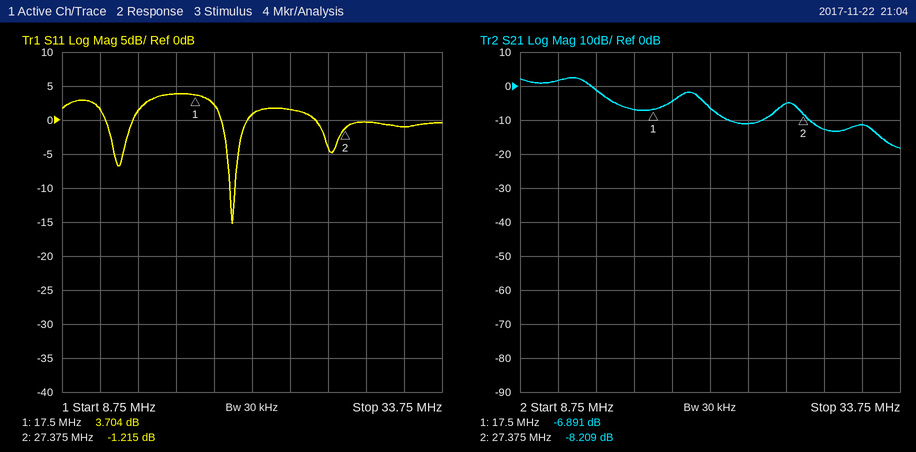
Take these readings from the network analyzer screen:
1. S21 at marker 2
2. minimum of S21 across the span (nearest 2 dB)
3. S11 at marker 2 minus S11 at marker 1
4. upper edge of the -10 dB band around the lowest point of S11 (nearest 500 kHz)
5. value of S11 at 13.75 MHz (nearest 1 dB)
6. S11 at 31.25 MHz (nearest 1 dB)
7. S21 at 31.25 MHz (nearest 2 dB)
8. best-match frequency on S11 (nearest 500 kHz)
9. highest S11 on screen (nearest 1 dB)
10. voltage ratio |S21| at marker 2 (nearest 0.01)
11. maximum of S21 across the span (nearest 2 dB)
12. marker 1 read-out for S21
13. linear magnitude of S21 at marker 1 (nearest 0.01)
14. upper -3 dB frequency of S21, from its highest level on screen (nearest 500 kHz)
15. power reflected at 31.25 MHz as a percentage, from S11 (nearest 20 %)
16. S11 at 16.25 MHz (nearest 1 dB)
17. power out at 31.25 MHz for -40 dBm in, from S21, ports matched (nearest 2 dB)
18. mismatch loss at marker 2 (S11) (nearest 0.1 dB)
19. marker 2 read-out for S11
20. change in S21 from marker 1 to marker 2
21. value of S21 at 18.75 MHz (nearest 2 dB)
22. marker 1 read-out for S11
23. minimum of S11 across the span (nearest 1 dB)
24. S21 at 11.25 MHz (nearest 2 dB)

-8.209 dB
-18 dB
-4.919 dB
20.0 MHz
1 dB
-1 dB
-12 dB
20.0 MHz
4 dB
0.39
2 dB
-6.891 dB
0.45
13.5 MHz
80 %
4 dB
-52 dBm
6.1 dB
-1.215 dB
-1.318 dB
-4 dB
3.704 dB
-15 dB
2 dB
